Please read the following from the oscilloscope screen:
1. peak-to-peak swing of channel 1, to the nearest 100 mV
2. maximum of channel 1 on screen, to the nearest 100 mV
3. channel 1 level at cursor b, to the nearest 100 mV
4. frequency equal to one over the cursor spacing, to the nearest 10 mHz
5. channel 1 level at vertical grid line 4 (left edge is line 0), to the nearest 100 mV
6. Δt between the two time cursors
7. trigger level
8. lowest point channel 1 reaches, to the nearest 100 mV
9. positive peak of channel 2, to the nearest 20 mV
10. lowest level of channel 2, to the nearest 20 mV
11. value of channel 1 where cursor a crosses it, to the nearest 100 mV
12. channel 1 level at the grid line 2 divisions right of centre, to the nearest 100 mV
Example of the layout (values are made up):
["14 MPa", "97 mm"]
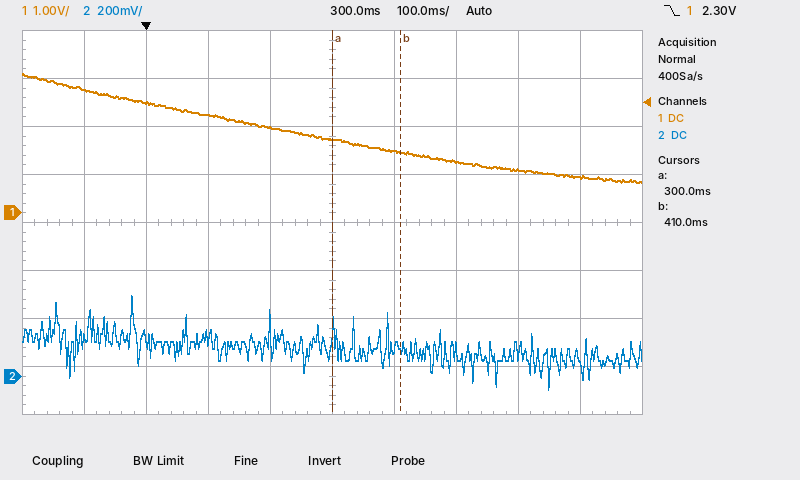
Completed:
["2.3 V", "2.9 V", "1.3 V", "9.09 Hz", "1.8 V", "110 ms", "2.30 V", "600 mV", "340 mV", "-60 mV", "1.5 V", "1.1 V"]
